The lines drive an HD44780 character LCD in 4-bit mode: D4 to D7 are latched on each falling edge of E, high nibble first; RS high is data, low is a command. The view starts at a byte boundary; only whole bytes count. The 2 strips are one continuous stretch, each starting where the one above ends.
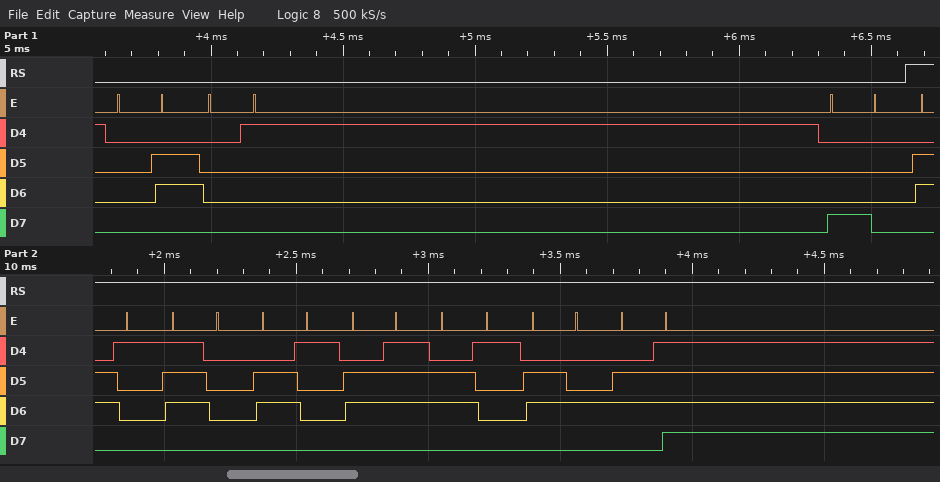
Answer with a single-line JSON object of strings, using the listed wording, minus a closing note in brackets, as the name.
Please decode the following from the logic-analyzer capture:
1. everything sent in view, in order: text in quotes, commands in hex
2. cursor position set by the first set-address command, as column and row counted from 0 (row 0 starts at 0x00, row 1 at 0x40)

{"everything sent in view, in order: text in quotes, commands in hex": "0x06 0x01 0x80 \"apagado\"", "cursor position set by the first set-address command, as column and row counted from 0": "column 0, row 0"}
